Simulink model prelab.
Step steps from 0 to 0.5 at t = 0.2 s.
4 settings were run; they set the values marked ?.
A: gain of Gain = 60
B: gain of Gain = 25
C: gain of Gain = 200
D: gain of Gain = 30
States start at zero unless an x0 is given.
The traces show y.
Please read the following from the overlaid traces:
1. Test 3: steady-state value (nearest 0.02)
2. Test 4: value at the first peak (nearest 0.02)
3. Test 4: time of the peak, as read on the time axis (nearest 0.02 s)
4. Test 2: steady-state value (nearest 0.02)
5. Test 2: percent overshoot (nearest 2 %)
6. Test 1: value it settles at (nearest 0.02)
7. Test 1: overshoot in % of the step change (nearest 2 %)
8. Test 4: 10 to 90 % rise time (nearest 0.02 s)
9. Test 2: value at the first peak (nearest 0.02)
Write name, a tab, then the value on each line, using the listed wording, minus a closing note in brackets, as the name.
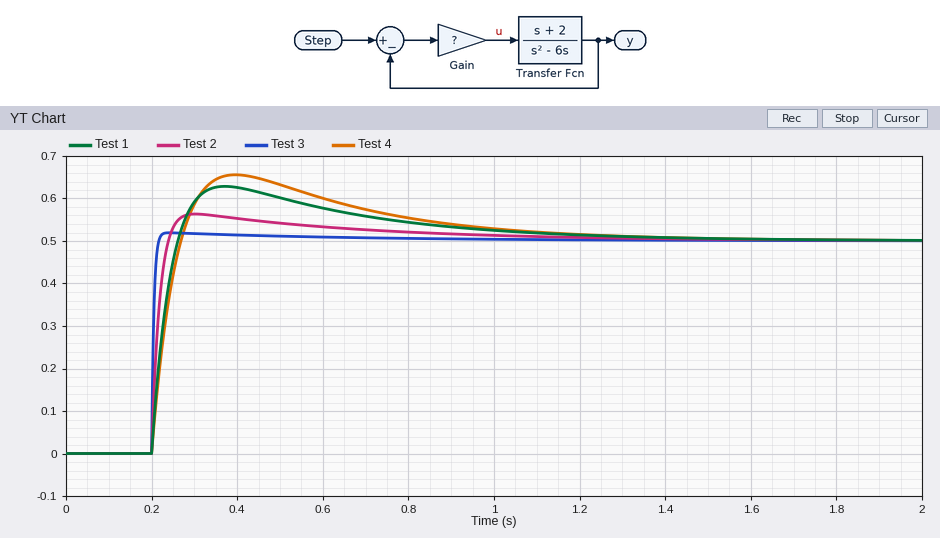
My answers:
Test 3: steady-state value	0.50
Test 4: value at the first peak	0.66
Test 4: time of the peak, as read on the time axis	0.40 s
Test 2: steady-state value	0.50
Test 2: percent overshoot	12 %
Test 1: value it settles at	0.50
Test 1: overshoot in % of the step change	26 %
Test 4: 10 to 90 % rise time	0.06 s
Test 2: value at the first peak	0.56
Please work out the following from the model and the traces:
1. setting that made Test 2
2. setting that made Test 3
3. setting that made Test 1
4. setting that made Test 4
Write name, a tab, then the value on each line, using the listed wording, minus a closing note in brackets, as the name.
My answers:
setting that made Test 2	A
setting that made Test 3	C
setting that made Test 1	D
setting that made Test 4	B
